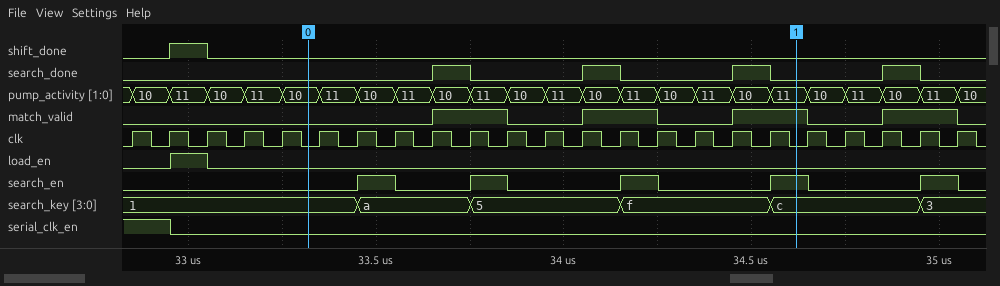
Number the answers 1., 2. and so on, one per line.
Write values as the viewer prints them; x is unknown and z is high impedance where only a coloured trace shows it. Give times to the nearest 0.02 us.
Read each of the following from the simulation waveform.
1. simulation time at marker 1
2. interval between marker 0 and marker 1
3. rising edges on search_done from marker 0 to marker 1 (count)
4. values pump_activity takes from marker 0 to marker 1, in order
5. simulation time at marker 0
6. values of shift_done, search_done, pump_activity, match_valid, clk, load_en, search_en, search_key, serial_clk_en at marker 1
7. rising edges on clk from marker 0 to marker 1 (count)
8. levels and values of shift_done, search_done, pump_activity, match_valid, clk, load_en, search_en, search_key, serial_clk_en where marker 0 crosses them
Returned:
1. 34.62 us
2. 1.3 us
3. 3
4. 10, 11, 10, 11, 10, 11, 10, 11, 10, 11, 10, 11, 10, 11
5. 33.32 us
6. shift_done=0, search_done=0, pump_activity=11, match_valid=1, clk=0, load_en=0, search_en=1, search_key=c, serial_clk_en=0
7. 13
8. shift_done=0, search_done=0, pump_activity=10, match_valid=0, clk=0, load_en=0, search_en=0, search_key=1, serial_clk_en=0
